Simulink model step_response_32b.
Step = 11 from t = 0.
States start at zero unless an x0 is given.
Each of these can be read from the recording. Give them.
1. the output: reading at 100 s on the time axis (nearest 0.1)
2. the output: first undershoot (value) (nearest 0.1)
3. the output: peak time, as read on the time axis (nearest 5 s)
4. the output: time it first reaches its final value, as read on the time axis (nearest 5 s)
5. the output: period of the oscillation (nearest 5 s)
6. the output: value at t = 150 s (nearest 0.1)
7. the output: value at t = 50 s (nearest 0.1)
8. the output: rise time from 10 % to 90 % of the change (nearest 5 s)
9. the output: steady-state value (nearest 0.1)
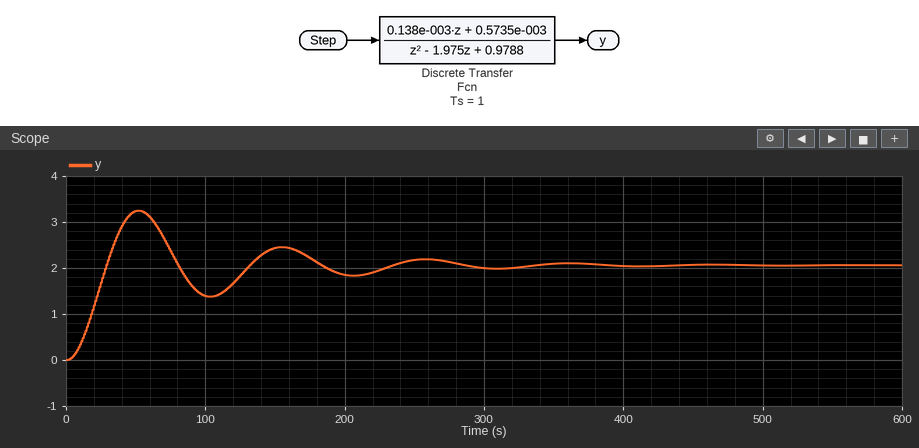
1.4
1.4
50 s
30 s
105 s
2.4
3.2
20 s
2.1
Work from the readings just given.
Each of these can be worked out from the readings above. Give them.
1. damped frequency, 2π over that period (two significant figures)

0.060 rad/s
